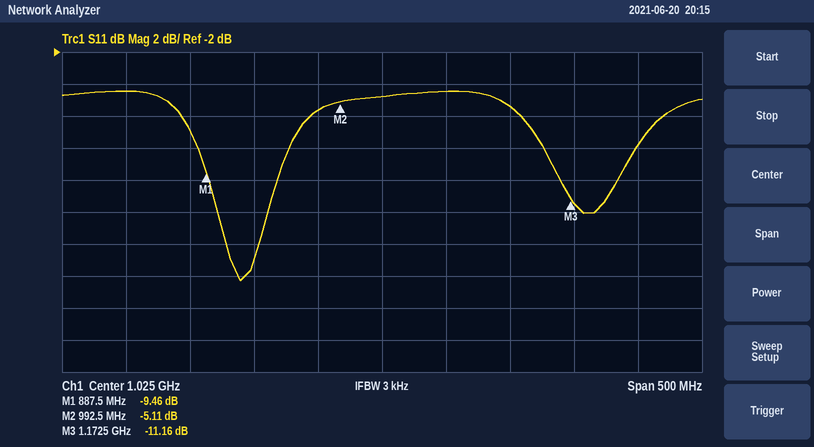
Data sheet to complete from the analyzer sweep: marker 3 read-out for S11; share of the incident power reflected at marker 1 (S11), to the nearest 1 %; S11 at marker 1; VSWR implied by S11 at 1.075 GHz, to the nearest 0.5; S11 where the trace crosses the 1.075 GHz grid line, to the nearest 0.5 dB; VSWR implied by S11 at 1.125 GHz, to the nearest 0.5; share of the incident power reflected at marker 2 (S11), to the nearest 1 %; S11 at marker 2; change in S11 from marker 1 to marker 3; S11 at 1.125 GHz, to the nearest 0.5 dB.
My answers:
-11.16 dB
11 %
-9.46 dB
4.0
-4.5 dB
3.5
31 %
-5.11 dB
-1.70 dB
-5.5 dB
